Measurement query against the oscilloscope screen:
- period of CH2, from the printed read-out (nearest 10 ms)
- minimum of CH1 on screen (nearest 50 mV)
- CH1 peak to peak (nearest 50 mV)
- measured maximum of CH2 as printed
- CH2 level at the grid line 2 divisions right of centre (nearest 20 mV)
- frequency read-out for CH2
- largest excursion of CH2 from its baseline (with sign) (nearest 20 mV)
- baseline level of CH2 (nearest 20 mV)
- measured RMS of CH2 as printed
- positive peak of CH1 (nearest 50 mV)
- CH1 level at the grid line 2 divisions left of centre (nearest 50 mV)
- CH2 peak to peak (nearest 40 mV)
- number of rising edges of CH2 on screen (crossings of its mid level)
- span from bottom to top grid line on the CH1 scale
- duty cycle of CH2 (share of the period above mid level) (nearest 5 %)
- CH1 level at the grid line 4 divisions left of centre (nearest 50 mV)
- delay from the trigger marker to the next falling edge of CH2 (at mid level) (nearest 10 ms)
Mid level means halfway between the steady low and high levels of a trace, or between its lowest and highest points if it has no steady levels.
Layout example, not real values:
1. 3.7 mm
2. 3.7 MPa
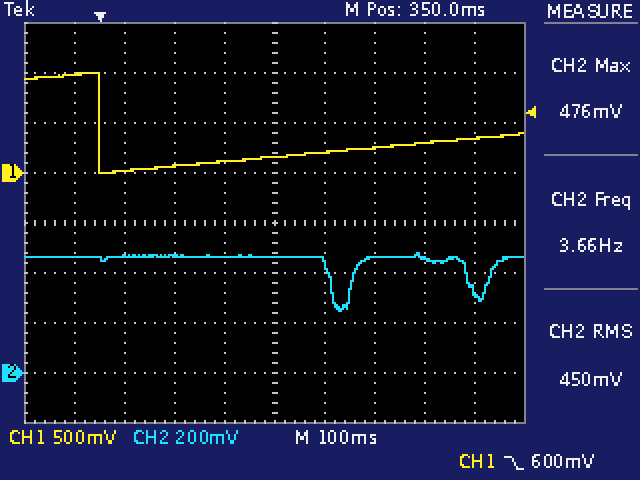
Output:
1. 270 ms
2. 0 mV
3. 1.00 V
4. 476 mV
5. 460 mV
6. 3.66 Hz
7. -220 mV
8. 460 mV
9. 450 mV
10. 1.00 V
11. 50 mV
12. 240 mV
13. 2
14. 4 V
15. 85 %
16. 1.00 V
17. 460 ms
